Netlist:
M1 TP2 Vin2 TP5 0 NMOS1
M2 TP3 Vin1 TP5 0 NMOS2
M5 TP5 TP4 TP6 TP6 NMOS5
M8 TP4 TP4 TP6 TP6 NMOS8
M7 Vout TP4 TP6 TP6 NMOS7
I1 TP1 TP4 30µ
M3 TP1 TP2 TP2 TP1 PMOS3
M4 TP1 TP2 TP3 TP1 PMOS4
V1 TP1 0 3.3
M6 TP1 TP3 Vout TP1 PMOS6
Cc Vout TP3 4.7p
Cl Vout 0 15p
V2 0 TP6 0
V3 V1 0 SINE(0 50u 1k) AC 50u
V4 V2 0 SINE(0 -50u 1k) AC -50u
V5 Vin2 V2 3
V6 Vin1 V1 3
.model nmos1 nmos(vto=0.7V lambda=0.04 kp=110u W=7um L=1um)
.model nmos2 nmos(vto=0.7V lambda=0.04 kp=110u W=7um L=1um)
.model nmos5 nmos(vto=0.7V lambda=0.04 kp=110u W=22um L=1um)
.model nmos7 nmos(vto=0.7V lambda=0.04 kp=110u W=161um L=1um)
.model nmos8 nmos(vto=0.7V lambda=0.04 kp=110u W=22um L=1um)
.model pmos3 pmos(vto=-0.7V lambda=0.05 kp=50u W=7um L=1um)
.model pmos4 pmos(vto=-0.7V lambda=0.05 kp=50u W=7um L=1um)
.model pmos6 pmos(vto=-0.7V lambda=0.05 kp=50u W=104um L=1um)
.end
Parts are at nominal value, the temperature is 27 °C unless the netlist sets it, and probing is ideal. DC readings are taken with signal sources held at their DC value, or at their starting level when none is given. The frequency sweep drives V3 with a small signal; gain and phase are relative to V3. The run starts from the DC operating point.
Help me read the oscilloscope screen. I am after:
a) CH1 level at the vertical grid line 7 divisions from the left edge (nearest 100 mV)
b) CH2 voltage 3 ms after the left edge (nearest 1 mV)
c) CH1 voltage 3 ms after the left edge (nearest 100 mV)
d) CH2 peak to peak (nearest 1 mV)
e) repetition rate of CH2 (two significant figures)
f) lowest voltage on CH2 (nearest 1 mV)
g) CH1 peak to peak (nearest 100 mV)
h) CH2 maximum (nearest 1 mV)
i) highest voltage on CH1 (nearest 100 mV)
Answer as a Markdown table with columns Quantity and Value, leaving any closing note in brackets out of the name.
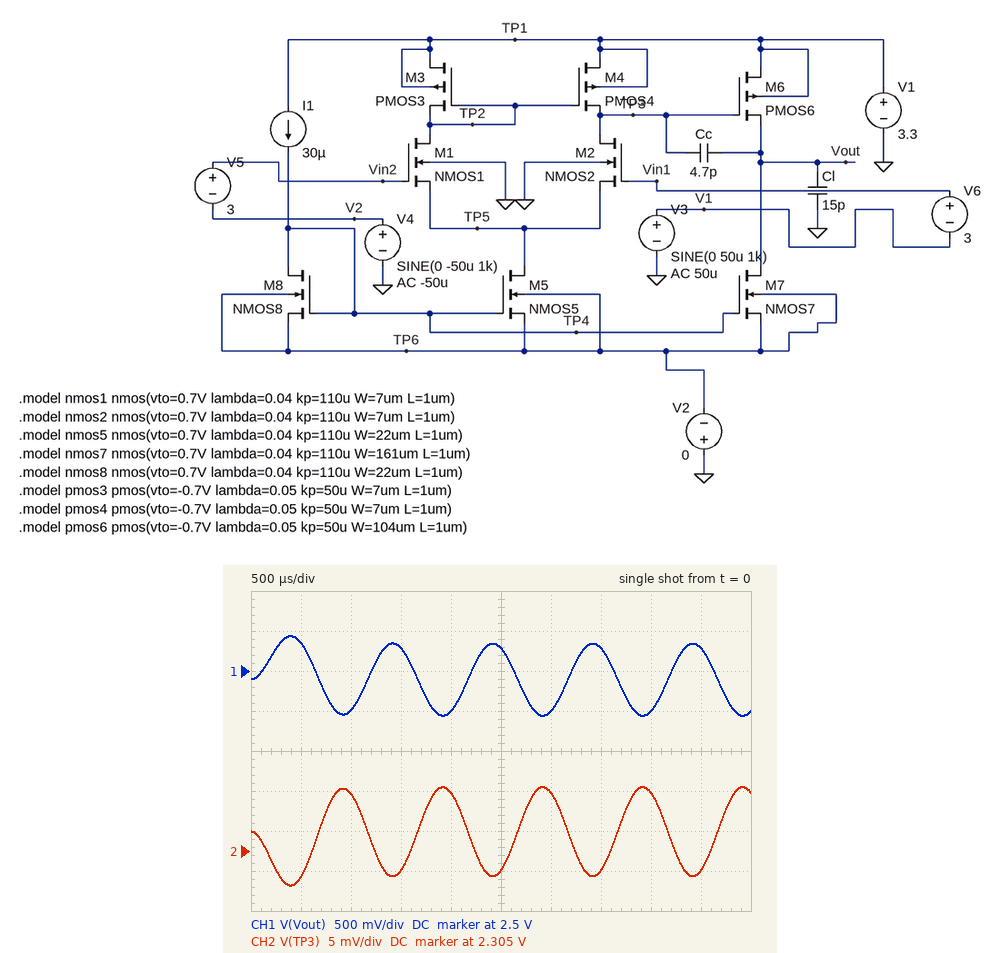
| Quantity | Value |
|---|---|
| CH1 level at the vertical grid line 7 divisions from the left edge | 2.8 V |
| CH2 voltage 3 ms after the left edge | 2.312 V |
| CH1 voltage 3 ms after the left edge | 2.0 V |
| CH2 peak to peak | 12 mV |
| repetition rate of CH2 | 1.0 kHz |
| lowest voltage on CH2 | 2.301 V |
| CH1 peak to peak | 1.0 V |
| CH2 maximum | 2.313 V |
| highest voltage on CH1 | 2.9 V |
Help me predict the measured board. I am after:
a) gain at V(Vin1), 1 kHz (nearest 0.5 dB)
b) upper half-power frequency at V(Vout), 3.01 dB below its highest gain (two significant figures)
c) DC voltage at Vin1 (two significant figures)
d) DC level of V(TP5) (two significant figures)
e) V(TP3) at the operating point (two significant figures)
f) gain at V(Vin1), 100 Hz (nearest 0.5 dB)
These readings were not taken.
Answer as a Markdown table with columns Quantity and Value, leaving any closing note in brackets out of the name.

| Quantity | Value |
|---|---|
| gain at V(Vin1), 1 kHz | 0 dB |
| upper half-power frequency at V(Vout), 3.01 dB below its highest gain | 560 Hz |
| DC voltage at Vin1 | 3.0 V |
| DC level of V(TP5) | 2.1 V |
| V(TP3) at the operating point | 2.3 V |
| gain at V(Vin1), 100 Hz | 0 dB |
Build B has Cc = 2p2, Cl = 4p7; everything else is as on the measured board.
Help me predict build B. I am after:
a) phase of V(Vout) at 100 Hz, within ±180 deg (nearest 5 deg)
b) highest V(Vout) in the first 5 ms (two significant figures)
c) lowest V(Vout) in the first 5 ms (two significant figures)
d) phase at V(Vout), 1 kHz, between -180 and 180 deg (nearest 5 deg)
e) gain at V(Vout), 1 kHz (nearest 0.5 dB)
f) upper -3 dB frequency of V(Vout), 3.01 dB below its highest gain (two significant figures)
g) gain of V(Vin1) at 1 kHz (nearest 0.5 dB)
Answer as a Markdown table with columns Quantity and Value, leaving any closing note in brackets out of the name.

| Quantity | Value |
|---|---|
| phase of V(Vout) at 100 Hz, within ±180 deg | -5 deg |
| highest V(Vout) in the first 5 ms | 3.0 V |
| lowest V(Vout) in the first 5 ms | 1.7 V |
| phase at V(Vout), 1 kHz, between -180 and 180 deg | -40 deg |
| gain at V(Vout), 1 kHz | 77.0 dB |
| upper -3 dB frequency of V(Vout), 3.01 dB below its highest gain | 1.2 kHz |
| gain of V(Vin1) at 1 kHz | 0 dB |
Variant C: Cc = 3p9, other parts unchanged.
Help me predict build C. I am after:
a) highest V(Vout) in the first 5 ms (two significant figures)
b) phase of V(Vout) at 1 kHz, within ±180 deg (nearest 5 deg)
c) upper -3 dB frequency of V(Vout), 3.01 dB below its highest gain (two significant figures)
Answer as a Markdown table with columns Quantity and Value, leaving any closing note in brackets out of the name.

| Quantity | Value |
|---|---|
| highest V(Vout) in the first 5 ms | 3.0 V |
| phase of V(Vout) at 1 kHz, within ±180 deg | -55 deg |
| upper -3 dB frequency of V(Vout), 3.01 dB below its highest gain | 680 Hz |
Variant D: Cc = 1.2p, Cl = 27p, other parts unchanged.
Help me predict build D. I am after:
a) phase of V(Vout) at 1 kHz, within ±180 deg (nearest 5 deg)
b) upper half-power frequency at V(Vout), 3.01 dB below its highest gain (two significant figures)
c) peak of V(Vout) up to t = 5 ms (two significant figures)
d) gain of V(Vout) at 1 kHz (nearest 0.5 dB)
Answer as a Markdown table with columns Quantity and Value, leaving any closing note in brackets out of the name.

| Quantity | Value |
|---|---|
| phase of V(Vout) at 1 kHz, within ±180 deg | -25 deg |
| upper half-power frequency at V(Vout), 3.01 dB below its highest gain | 2.2 kHz |
| peak of V(Vout) up to t = 5 ms | 3.0 V |
| gain of V(Vout) at 1 kHz | 78.5 dB |
